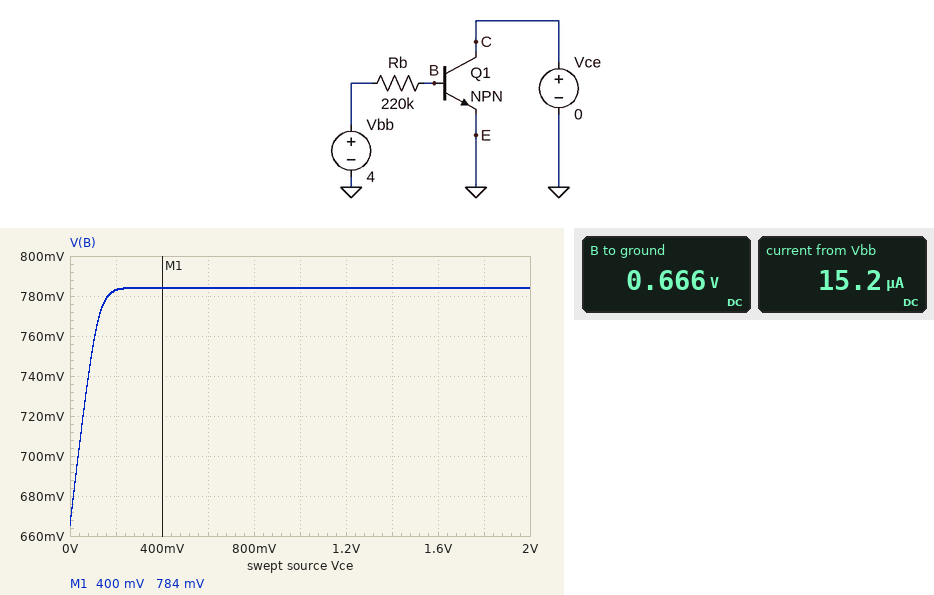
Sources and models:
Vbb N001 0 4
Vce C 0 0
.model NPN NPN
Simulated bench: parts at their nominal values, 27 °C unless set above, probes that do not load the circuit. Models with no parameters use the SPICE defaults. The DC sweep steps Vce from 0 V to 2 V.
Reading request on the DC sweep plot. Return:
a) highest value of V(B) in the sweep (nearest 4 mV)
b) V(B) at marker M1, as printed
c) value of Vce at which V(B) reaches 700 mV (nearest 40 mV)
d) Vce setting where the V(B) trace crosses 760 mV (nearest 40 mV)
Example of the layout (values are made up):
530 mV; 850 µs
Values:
784 mV; 784 mV; 40 mV; 120 mV
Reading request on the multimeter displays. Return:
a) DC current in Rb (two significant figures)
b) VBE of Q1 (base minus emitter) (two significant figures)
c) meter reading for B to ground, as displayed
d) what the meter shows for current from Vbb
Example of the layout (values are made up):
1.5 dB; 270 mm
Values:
15 µA; 670 mV; 0.666 V; 15.2 µA
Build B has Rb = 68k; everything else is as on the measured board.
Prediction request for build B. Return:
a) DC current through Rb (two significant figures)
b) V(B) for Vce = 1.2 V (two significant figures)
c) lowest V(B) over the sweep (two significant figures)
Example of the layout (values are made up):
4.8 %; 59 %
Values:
49 µA; 810 mV; 700 mV
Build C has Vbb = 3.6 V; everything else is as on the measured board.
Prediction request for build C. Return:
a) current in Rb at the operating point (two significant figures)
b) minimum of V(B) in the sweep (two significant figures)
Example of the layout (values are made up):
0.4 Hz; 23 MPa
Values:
13 µA; 660 mV
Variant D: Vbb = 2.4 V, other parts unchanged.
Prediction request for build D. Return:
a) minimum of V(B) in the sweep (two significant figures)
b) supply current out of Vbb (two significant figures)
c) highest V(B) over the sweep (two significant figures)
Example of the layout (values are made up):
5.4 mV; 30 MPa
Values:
650 mV; 8.0 µA; 770 mV
